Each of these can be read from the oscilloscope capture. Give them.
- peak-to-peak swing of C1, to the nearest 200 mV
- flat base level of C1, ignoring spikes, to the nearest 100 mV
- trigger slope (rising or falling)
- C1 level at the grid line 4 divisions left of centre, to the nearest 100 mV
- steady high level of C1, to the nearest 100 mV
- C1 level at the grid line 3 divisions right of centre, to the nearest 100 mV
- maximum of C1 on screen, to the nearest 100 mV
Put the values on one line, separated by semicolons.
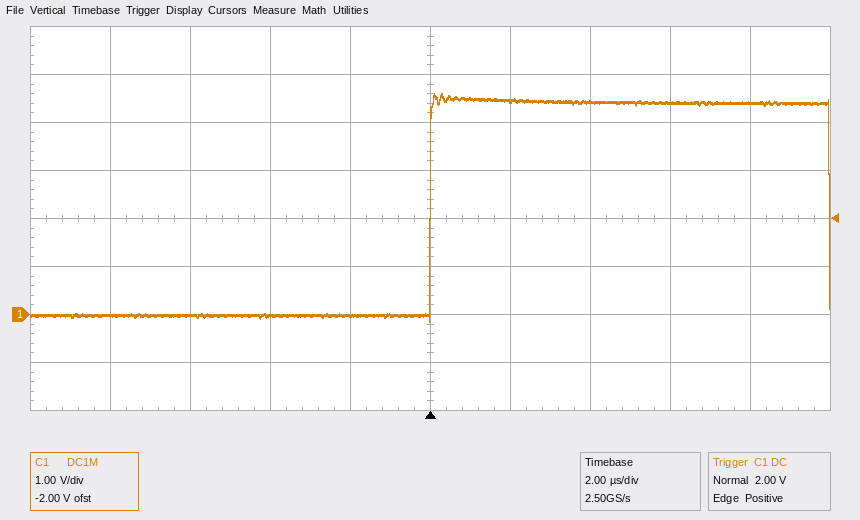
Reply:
4.8 V; 0.0 V; rising; 0.0 V; 4.4 V; 4.4 V; 4.6 V
